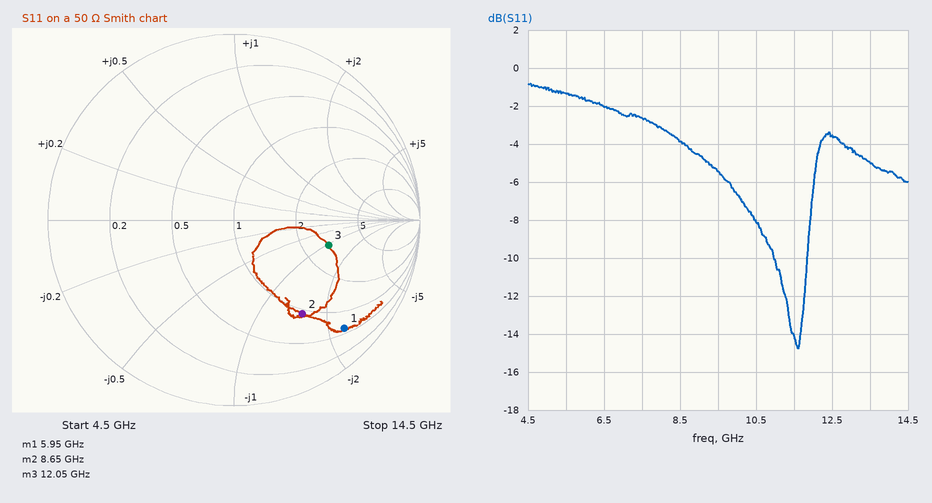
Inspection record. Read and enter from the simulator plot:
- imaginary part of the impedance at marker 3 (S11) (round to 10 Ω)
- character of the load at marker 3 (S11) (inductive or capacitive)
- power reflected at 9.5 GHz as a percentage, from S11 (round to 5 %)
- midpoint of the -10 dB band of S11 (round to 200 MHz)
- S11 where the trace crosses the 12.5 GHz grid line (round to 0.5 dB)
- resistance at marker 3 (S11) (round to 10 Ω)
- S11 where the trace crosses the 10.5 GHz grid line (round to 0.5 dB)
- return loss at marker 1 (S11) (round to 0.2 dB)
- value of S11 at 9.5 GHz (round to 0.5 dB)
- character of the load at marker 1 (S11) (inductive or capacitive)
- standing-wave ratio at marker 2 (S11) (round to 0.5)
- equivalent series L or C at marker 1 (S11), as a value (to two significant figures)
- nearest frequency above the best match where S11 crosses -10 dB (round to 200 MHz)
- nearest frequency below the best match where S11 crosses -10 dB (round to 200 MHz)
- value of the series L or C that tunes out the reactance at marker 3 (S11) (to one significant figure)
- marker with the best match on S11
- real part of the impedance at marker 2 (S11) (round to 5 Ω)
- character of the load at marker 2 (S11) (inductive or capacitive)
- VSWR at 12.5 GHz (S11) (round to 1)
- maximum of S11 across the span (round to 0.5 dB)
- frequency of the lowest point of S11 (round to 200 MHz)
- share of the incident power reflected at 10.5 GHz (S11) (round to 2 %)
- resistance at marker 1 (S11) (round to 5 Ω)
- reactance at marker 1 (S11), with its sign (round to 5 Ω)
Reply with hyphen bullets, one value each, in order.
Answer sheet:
- -50 Ω
- capacitive
- 30 %
- 11.4 GHz
- -3.5 dB
- 140 Ω
- -8.0 dB
- 1.6 dB
- -5.5 dB
- capacitive
- 4.5
- 230 fF
- 11.8 GHz
- 11.0 GHz
- 700 pH
- marker 3
- 45 Ω
- capacitive
- 5
- -1.0 dB
- 11.6 GHz
- 16 %
- 30 Ω
- -115 Ω
